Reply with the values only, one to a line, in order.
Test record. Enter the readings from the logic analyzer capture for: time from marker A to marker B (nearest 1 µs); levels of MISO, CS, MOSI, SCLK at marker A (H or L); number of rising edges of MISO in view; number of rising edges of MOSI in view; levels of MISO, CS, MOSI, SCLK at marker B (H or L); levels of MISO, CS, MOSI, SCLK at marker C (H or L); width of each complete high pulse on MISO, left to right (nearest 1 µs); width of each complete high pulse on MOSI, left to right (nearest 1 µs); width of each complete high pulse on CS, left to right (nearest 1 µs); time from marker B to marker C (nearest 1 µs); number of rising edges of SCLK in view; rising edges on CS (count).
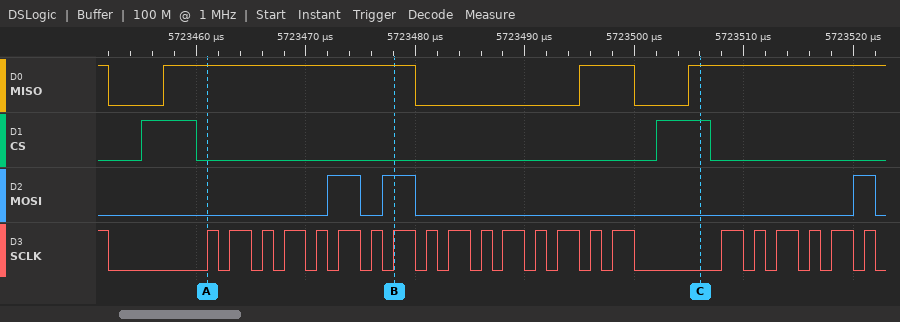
17 µs
MISO=H, CS=L, MOSI=L, SCLK=H
3
3
MISO=H, CS=L, MOSI=H, SCLK=H
MISO=H, CS=H, MOSI=L, SCLK=L
23 µs, 5 µs
3 µs, 3 µs, 2 µs
5 µs, 5 µs
28 µs
22
2
